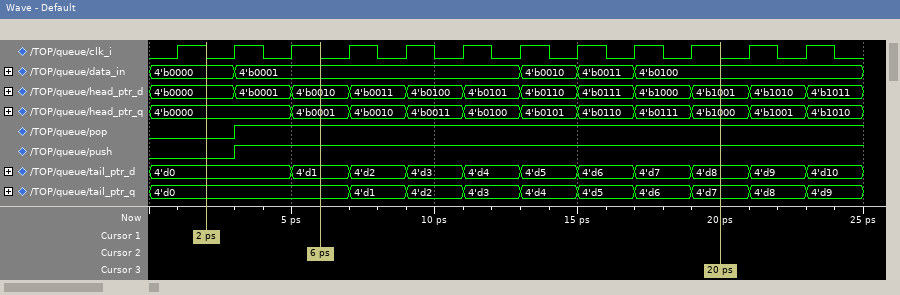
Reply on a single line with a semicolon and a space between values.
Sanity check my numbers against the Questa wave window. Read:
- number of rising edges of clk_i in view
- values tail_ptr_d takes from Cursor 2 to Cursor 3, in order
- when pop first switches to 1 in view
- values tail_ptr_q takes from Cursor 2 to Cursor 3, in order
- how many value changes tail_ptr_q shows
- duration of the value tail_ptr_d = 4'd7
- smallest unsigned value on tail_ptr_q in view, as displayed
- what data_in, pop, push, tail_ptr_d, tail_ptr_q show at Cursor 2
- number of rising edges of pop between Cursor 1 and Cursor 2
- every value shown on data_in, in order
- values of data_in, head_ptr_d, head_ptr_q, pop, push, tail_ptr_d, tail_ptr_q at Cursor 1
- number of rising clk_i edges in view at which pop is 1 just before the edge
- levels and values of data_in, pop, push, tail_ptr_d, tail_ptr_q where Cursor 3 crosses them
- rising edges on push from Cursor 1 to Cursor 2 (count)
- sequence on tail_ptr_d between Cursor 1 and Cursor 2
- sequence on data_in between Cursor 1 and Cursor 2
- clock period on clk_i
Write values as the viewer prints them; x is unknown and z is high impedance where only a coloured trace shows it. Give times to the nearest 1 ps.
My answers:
12; 4'd1, 4'd2, 4'd3, 4'd4, 4'd5, 4'd6, 4'd7, 4'd8; 3 ps; 4'd0, 4'd1, 4'd2, 4'd3, 4'd4, 4'd5, 4'd6, 4'd7; 9; 2 ps; 4'd0; data_in=4'b0001, pop=1, push=1, tail_ptr_d=4'd1, tail_ptr_q=4'd0; 1; 4'b0000, 4'b0001, 4'b0010, 4'b0011, 4'b0100; data_in=4'b0000, head_ptr_d=4'b0000, head_ptr_q=4'b0000, pop=0, push=0, tail_ptr_d=4'd0, tail_ptr_q=4'd0; 10; data_in=4'b0100, pop=1, push=1, tail_ptr_d=4'd8, tail_ptr_q=4'd7; 1; 4'd0, 4'd1; 4'b0000, 4'b0001; 2 ps
